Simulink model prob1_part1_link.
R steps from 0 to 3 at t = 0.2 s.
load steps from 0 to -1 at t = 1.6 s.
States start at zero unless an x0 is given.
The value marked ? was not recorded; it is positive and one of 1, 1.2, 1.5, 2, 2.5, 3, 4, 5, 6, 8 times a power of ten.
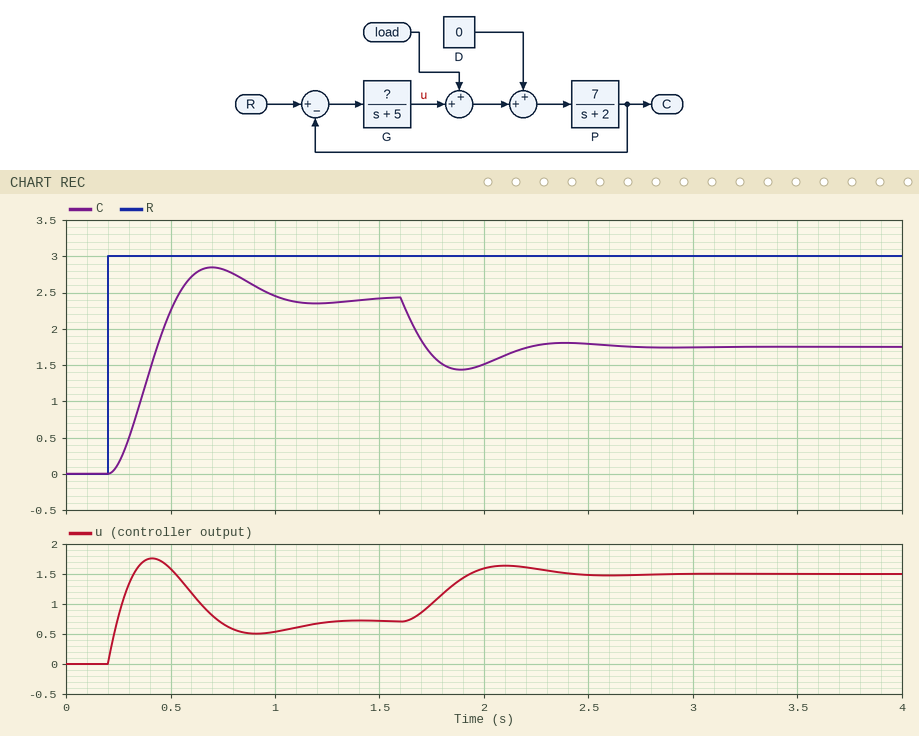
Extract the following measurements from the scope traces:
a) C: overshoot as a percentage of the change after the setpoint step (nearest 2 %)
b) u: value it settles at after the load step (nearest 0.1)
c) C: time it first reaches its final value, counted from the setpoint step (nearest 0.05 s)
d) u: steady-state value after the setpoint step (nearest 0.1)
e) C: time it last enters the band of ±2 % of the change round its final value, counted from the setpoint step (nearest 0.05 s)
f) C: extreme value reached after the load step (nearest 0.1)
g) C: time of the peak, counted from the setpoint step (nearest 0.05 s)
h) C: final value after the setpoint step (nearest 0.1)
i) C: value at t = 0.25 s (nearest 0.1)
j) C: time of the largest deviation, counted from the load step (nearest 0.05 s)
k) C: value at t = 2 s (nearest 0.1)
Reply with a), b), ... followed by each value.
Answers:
a) 18 %
b) 1.5
c) 0.35 s
d) 0.7
e) 1.15 s
f) 1.4
g) 0.50 s
h) 2.4
i) 0.1
j) 0.30 s
k) 1.5
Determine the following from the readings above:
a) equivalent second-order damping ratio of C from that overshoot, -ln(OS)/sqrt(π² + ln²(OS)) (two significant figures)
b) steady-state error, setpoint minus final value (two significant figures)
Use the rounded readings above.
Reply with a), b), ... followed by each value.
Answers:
a) 0.48
b) 0.60
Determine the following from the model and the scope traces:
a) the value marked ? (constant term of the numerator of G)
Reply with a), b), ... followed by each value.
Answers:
a) 6
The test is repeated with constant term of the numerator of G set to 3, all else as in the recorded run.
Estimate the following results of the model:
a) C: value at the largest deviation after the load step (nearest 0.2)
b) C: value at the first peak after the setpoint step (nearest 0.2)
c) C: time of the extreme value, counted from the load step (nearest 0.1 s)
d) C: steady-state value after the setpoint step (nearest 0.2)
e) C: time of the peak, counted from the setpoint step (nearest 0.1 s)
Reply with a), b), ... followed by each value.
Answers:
a) 0.6
b) 2.2
c) 0.4 s
d) 2.0
e) 0.7 s
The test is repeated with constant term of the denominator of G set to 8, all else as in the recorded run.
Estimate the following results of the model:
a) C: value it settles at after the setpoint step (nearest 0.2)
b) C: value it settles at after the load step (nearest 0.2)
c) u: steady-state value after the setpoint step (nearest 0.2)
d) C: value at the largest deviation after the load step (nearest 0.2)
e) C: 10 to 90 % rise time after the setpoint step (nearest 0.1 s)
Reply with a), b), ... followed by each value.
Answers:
a) 2.2
b) 1.2
c) 0.6
d) 1.0
e) 0.3 s
